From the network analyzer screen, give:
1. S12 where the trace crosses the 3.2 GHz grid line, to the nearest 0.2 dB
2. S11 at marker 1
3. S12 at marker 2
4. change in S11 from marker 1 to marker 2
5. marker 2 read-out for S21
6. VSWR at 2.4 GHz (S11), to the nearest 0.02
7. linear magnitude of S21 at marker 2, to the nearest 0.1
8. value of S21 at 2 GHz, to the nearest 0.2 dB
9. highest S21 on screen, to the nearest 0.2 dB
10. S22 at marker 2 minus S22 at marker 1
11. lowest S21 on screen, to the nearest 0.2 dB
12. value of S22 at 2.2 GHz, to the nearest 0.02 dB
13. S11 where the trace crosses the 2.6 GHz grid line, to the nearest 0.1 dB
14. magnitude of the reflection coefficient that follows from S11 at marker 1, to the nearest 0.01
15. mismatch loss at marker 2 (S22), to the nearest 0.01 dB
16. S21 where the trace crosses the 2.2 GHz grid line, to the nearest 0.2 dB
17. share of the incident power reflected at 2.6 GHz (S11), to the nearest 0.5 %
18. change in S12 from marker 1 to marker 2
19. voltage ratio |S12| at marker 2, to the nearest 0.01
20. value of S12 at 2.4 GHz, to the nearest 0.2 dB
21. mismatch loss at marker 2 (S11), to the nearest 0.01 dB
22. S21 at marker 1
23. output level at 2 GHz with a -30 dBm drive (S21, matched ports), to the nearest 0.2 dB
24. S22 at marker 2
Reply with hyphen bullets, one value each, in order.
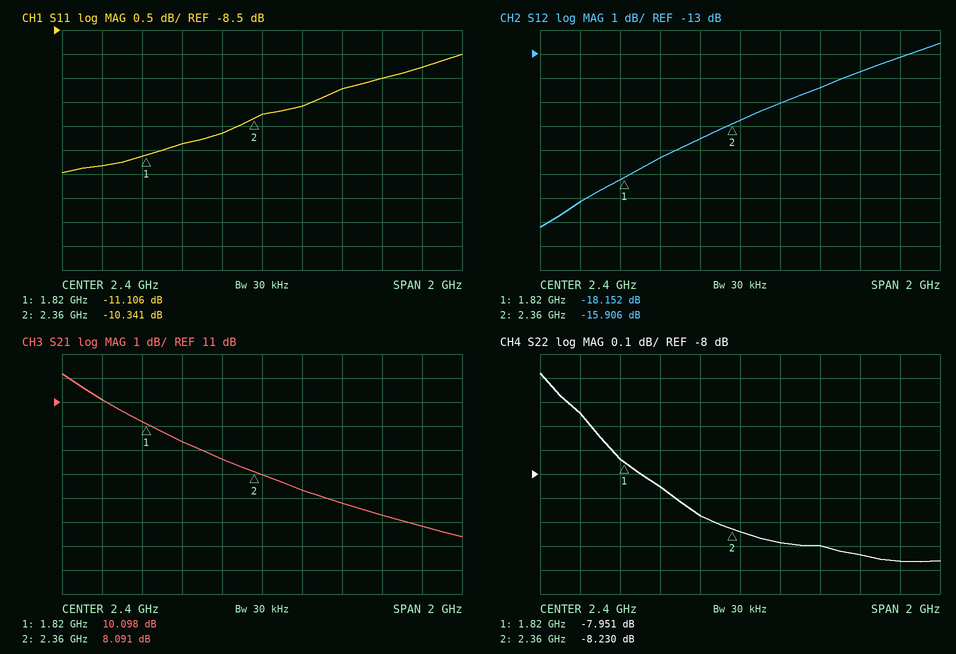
- -13.2 dB
- -11.106 dB
- -15.906 dB
- 0.765 dB
- 8.091 dB
- 1.88
- 2.5
- 9.4 dB
- 12.2 dB
- -0.279 dB
- 5.4 dB
- -8.18 dB
- -10.1 dB
- 0.28
- 0.71 dB
- 8.6 dB
- 10.0 %
- 2.246 dB
- 0.16
- -15.8 dB
- 0.42 dB
- 10.098 dB
- -20.6 dBm
- -8.230 dB
